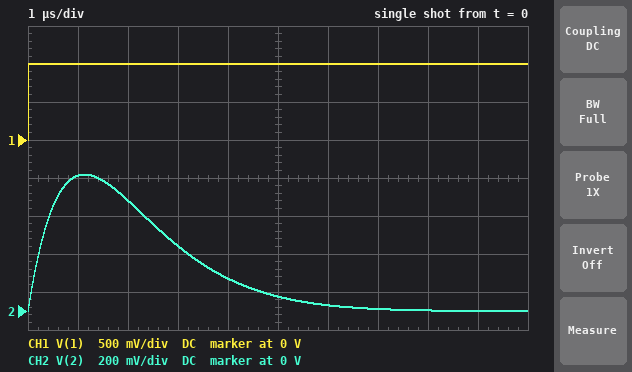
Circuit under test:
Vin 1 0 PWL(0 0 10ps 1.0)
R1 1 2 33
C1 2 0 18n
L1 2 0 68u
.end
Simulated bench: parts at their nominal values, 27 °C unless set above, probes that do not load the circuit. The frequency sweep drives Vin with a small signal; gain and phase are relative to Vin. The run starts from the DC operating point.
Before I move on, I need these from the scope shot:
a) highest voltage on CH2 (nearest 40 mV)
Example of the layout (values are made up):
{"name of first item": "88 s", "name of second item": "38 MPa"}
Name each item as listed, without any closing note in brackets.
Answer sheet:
{"highest voltage on CH2": "720 mV"}
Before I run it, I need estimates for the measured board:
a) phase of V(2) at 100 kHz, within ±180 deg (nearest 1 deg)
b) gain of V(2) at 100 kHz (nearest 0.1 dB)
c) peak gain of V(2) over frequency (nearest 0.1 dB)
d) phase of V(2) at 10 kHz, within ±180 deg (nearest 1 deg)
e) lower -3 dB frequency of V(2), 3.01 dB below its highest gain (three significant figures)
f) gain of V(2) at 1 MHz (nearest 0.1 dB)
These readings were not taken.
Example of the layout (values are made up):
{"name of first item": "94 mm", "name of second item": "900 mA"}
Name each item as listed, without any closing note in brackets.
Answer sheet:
{"phase of V(2) at 100 kHz, within ±180 deg": "22 deg", "gain of V(2) at 100 kHz": "-0.6 dB", "peak gain of V(2) over frequency": "0 dB", "phase of V(2) at 10 kHz, within ±180 deg": "83 deg", "lower -3 dB frequency of V(2), 3.01 dB below its highest gain": "62.6 kHz", "gain of V(2) at 1 MHz": "-11.6 dB"}
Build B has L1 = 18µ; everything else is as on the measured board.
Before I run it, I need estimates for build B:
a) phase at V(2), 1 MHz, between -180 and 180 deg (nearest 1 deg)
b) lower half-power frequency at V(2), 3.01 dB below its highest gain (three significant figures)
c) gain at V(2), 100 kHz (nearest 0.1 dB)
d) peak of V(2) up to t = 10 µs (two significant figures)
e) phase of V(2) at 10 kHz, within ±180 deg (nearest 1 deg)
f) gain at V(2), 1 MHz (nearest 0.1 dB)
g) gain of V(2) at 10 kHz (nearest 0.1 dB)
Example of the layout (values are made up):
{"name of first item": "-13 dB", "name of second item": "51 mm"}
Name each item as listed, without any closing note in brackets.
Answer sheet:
{"phase at V(2), 1 MHz, between -180 and 180 deg": "-74 deg", "lower half-power frequency at V(2), 3.01 dB below its highest gain": "176 kHz", "gain at V(2), 100 kHz": "-8.7 dB", "peak of V(2) up to t = 10 µs": "530 mV", "phase of V(2) at 10 kHz, within ±180 deg": "88 deg", "gain at V(2), 1 MHz": "-11.1 dB", "gain of V(2) at 10 kHz": "-29.3 dB"}
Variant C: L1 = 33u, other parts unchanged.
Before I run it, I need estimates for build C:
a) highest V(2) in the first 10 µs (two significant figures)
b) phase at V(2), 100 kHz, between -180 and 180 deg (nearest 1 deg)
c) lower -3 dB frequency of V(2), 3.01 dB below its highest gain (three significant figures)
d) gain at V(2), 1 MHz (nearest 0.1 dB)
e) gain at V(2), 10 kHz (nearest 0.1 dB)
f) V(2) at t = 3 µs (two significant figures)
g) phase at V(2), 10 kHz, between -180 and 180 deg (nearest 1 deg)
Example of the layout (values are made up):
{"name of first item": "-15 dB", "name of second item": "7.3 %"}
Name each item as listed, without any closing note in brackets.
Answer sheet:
{"highest V(2) in the first 10 µs": "620 mV", "phase at V(2), 100 kHz, between -180 and 180 deg": "51 deg", "lower -3 dB frequency of V(2), 3.01 dB below its highest gain": "112 kHz", "gain at V(2), 1 MHz": "-11.4 dB", "gain at V(2), 10 kHz": "-24.0 dB", "V(2) at t = 3 µs": "24 mV", "phase at V(2), 10 kHz, between -180 and 180 deg": "86 deg"}
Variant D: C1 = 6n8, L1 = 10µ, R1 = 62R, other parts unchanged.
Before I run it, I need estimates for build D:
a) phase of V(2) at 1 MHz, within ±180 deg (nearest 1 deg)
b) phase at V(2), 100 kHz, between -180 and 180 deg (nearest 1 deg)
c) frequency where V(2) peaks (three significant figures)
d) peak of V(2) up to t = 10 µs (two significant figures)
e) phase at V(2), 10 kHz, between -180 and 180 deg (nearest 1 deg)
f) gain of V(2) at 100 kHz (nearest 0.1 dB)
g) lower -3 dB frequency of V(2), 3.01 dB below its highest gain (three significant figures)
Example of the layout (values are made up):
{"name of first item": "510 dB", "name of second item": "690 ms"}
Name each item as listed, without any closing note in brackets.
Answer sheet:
{"phase of V(2) at 1 MHz, within ±180 deg": "-59 deg", "phase at V(2), 100 kHz, between -180 and 180 deg": "84 deg", "frequency where V(2) peaks": "610 kHz", "peak of V(2) up to t = 10 µs": "410 mV", "phase at V(2), 10 kHz, between -180 and 180 deg": "89 deg", "gain of V(2) at 100 kHz": "-19.7 dB", "lower -3 dB frequency of V(2), 3.01 dB below its highest gain": "450 kHz"}
